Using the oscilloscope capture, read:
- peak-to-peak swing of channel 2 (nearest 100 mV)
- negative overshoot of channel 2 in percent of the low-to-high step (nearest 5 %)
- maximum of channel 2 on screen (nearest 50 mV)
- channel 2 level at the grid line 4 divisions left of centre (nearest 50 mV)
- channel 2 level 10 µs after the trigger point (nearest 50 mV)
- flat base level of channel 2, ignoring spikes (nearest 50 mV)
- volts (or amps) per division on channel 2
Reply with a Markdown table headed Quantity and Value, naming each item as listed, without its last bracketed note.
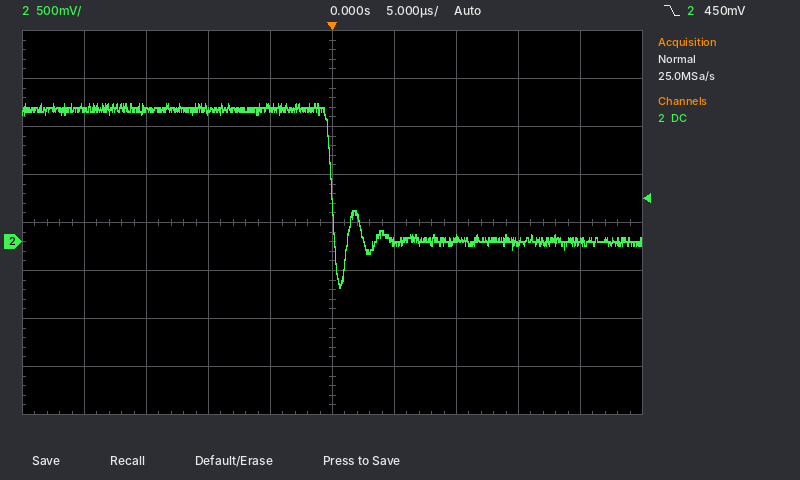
| Quantity | Value |
|---|---|
| peak-to-peak swing of channel 2 | 1.90 V |
| negative overshoot of channel 2 in percent of the low-to-high step | 35 % |
| maximum of channel 2 on screen | 1.45 V |
| channel 2 level at the grid line 4 divisions left of centre | 1.40 V |
| channel 2 level 10 µs after the trigger point | 50 mV |
| flat base level of channel 2, ignoring spikes | 0 mV |
| volts (or amps) per division on channel 2 | 500 mV |
